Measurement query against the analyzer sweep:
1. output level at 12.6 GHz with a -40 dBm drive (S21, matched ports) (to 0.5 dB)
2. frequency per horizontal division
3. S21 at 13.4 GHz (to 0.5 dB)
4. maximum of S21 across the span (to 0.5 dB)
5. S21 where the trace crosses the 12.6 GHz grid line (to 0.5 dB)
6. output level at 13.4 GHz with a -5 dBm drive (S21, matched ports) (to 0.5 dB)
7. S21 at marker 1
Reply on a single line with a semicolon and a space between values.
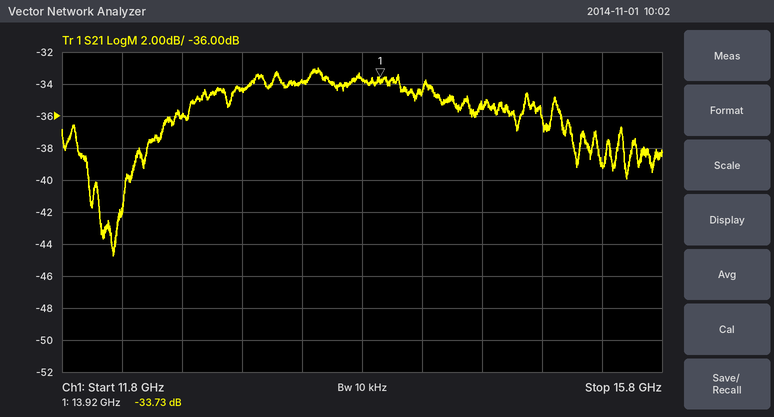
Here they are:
-76.0 dBm; 400 MHz; -34.0 dB; -33.0 dB; -36.0 dB; -39.0 dBm; -33.73 dB
